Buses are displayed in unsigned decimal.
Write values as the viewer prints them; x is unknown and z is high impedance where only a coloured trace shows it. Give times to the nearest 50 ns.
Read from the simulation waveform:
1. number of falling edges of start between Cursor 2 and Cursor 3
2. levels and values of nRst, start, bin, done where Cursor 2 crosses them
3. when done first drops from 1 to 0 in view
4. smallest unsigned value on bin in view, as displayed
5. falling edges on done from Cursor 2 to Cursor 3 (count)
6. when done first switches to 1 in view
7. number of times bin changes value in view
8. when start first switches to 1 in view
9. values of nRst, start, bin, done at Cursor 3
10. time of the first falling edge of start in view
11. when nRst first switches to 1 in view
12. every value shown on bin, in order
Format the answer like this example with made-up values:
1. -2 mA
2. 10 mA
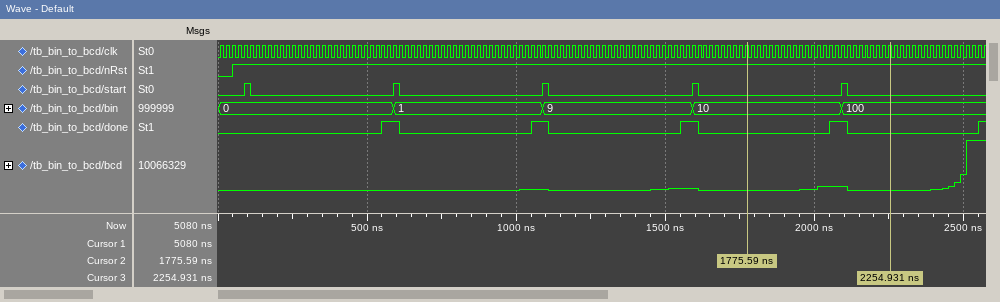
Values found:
1. 1
2. nRst=1, start=0, bin=10, done=0
3. 600 ns
4. 0
5. 1
6. 550 ns
7. 4
8. 100 ns
9. nRst=1, start=0, bin=100, done=0
10. 100 ns
11. 50 ns
12. 0, 1, 9, 10, 100
